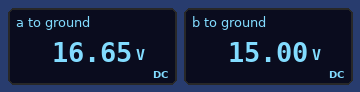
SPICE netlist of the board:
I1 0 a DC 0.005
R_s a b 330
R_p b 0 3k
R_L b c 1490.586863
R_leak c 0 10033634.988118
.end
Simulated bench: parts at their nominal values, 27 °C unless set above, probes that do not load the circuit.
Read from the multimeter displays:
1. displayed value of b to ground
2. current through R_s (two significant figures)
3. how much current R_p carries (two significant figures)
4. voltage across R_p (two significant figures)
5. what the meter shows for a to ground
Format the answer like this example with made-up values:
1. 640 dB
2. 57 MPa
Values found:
1. 15.00 V
2. 5.0 mA
3. 5.0 mA
4. 15 V
5. 16.65 V
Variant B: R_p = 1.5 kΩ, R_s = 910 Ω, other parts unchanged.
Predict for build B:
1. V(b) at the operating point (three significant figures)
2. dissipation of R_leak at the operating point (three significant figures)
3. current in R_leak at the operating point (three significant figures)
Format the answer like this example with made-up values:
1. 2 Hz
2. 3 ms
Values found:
1. 7.50 V
2. 5.60 µW
3. 747 nA
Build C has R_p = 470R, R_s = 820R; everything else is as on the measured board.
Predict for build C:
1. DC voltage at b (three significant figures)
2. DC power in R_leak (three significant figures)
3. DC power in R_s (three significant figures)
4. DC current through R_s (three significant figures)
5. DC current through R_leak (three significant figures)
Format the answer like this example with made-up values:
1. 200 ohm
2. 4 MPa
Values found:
1. 2.35 V
2. 550 nW
3. 20.5 mW
4. 5.00 mA
5. 234 nA
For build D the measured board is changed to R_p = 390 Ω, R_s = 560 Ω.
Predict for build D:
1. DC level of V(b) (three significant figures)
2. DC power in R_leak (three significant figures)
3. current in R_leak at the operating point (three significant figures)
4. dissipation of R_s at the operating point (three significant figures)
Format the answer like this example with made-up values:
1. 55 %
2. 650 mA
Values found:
1. 1.95 V
2. 379 nW
3. 194 nA
4. 14.0 mW
